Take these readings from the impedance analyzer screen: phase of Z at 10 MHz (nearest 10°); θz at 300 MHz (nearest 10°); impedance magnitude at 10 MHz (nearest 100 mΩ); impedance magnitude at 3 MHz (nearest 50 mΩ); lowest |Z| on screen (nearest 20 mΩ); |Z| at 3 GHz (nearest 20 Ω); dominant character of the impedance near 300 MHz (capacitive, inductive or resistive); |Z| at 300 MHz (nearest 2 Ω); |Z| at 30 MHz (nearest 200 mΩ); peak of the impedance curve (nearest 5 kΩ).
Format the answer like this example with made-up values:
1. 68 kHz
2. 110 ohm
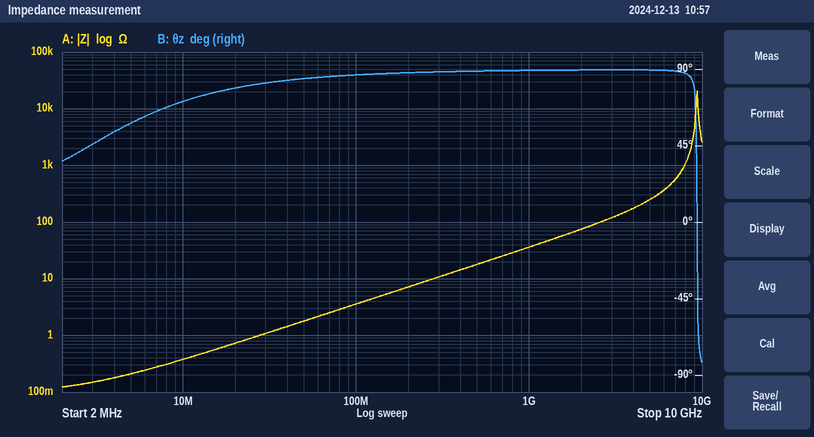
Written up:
1. 70°
2. 90°
3. 400 mΩ
4. 150 mΩ
5. 120 mΩ
6. 120 Ω
7. inductive
8. 10 Ω
9. 1.0 Ω
10. 20 kΩ
